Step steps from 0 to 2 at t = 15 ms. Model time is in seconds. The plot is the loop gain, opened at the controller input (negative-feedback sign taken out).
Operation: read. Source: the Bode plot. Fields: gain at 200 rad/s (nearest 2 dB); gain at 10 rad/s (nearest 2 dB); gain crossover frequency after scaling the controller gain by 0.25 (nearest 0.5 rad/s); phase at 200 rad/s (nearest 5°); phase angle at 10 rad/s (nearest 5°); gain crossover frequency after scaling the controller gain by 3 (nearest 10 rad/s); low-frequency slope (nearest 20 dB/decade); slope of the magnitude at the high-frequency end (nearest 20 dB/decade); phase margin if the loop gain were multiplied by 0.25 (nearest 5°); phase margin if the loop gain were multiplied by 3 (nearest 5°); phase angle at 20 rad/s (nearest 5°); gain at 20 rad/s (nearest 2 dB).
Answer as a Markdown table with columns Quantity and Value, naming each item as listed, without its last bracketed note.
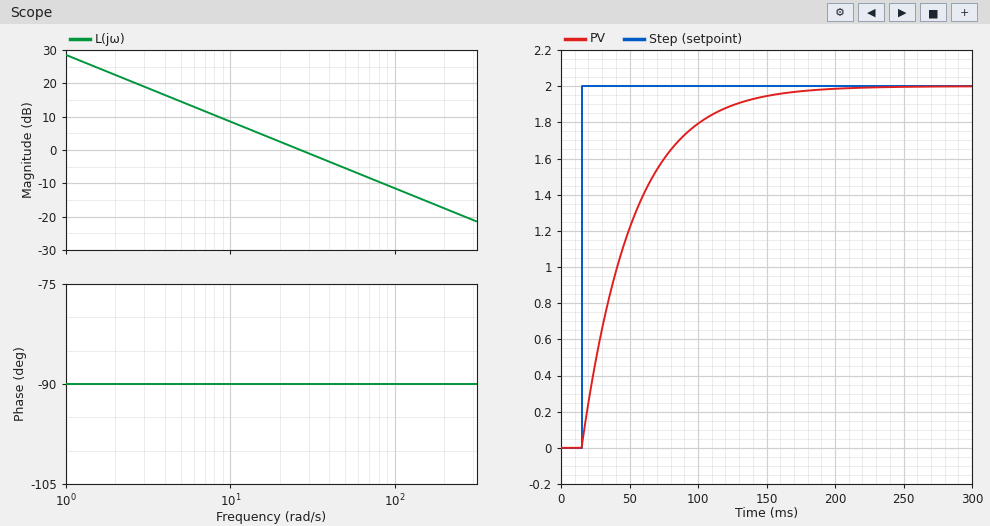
| Quantity | Value |
|---|---|
| gain at 200 rad/s | -18 dB |
| gain at 10 rad/s | 8 dB |
| gain crossover frequency after scaling the controller gain by 0.25 | 6.5 rad/s |
| phase at 200 rad/s | -90° |
| phase angle at 10 rad/s | -90° |
| gain crossover frequency after scaling the controller gain by 3 | 80 rad/s |
| low-frequency slope | -20 dB/decade |
| slope of the magnitude at the high-frequency end | -20 dB/decade |
| phase margin if the loop gain were multiplied by 0.25 | 90° |
| phase margin if the loop gain were multiplied by 3 | 90° |
| phase angle at 20 rad/s | -90° |
| gain at 20 rad/s | 2 dB |
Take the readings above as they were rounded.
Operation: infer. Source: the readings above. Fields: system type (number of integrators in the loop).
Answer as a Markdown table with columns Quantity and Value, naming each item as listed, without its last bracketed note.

| Quantity | Value |
|---|---|
| system type | 1 |
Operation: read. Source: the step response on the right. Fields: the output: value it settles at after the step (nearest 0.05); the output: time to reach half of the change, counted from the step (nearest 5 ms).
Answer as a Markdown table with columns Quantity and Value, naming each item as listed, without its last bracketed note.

| Quantity | Value |
|---|---|
| the output: value it settles at after the step | 2.00 |
| the output: time to reach half of the change, counted from the step | 25 ms |
